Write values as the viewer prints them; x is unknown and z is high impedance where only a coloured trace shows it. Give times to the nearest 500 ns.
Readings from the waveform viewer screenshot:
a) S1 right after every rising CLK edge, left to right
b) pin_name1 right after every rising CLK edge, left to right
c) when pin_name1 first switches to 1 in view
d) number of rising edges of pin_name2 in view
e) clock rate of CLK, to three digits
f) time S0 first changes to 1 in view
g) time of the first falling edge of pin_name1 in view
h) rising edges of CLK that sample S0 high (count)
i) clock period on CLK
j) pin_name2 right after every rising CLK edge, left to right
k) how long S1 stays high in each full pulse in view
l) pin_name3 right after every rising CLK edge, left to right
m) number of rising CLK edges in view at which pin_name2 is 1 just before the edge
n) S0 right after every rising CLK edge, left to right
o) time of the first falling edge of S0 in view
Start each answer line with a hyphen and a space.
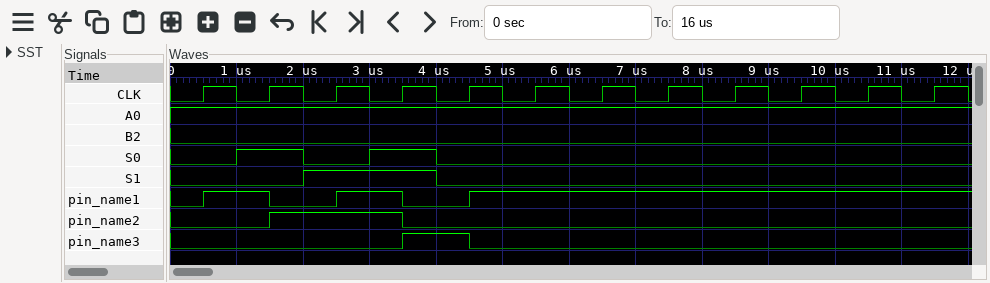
- 0 0 1 1 0 0 0 0 0 0 0 0
- 1 0 1 0 1 1 1 1 1 1 1 1
- 500 ns
- 1
- 1.00 MHz
- 1000 ns
- 1500 ns
- 2
- 1000 ns
- 0 1 1 0 0 0 0 0 0 0 0 0
- 2000 ns
- 0 0 0 1 0 0 0 0 0 0 0 0
- 2
- 0 1 0 1 0 0 0 0 0 0 0 0
- 2000 ns
